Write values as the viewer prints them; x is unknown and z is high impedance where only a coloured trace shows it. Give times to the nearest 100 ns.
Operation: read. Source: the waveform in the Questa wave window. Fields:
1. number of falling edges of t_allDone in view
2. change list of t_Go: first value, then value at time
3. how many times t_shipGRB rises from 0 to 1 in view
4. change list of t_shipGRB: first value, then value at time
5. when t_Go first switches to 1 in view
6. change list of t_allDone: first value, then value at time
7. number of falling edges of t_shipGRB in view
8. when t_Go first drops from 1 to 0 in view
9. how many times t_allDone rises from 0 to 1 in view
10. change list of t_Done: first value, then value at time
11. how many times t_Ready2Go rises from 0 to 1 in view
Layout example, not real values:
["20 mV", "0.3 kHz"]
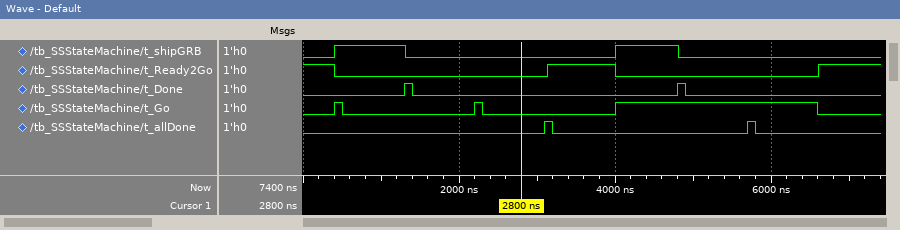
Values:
["2", "0, 1 at 400 ns, 0 at 500 ns, 1 at 2200 ns, 0 at 2300 ns, 1 at 4000 ns, 0 at 6600 ns", "2", "0, 1 at 400 ns, 0 at 1300 ns, 1 at 4000 ns, 0 at 4800 ns", "400 ns", "0, 1 at 3100 ns, 0 at 3200 ns, 1 at 5700 ns, 0 at 5800 ns", "2", "500 ns", "2", "0, 1 at 1300 ns, 0 at 1400 ns, 1 at 4800 ns, 0 at 4900 ns", "2"]
